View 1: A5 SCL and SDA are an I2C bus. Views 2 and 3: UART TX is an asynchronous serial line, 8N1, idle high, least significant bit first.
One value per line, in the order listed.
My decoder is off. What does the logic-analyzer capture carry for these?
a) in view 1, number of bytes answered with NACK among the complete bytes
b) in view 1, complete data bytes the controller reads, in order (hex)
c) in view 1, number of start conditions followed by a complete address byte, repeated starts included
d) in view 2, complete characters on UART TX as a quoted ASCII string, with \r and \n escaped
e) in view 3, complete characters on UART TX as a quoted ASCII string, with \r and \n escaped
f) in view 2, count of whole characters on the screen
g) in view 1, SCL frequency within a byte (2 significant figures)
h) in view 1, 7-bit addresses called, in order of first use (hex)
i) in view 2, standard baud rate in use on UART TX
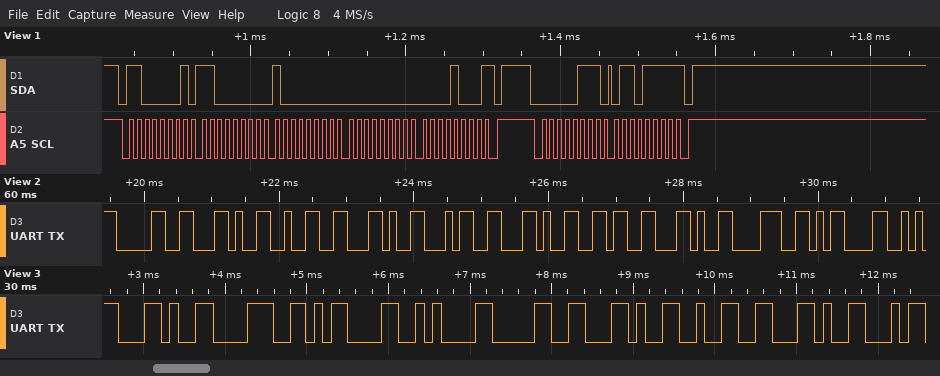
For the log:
2
C0 80 00 08 6F
2
"0,2,4,6,8\r"
",8\r\n0,2,"
10
100 kHz
0x60 0x03
9600 baud
